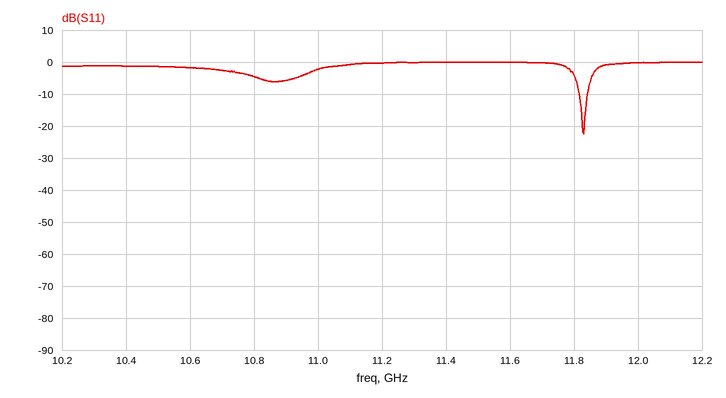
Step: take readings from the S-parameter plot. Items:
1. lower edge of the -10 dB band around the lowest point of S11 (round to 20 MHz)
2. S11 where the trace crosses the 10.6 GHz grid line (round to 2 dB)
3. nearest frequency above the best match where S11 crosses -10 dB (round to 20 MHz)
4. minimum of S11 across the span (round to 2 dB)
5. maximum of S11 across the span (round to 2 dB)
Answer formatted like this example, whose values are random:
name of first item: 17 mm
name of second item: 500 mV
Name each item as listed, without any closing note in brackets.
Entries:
lower edge of the -10 dB band around the lowest point of S11: 11.82 GHz
S11 where the trace crosses the 10.6 GHz grid line: -2 dB
nearest frequency above the best match where S11 crosses -10 dB: 11.84 GHz
minimum of S11 across the span: -22 dB
maximum of S11 across the span: 0 dB
